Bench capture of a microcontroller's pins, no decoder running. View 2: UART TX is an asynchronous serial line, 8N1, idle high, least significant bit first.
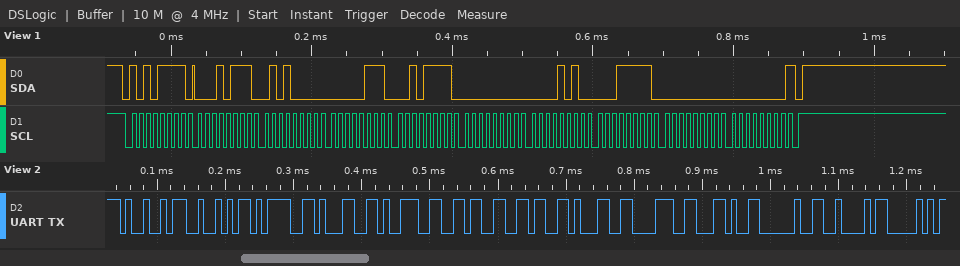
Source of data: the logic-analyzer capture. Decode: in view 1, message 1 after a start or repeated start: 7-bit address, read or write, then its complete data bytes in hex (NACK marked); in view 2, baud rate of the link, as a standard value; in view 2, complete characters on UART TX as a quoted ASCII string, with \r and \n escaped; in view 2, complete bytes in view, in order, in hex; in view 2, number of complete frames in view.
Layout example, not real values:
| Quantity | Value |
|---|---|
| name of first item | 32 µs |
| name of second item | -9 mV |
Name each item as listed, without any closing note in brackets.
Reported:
| Quantity | Value |
|---|---|
| in view 1, message 1 after a start or repeated start: 7-bit address, read or write, then its complete data bytes in hex | 0x57 read: 17 50 07 2F 00 0A 1F 00 00 NACK |
| in view 2, baud rate of the link, as a standard value | 115200 baud |
| in view 2, complete characters on UART TX as a quoted ASCII string, with \r and \n escaped | "IR=196618, BP" |
| in view 2, complete bytes in view, in order, in hex | 49 52 3D 31 39 36 36 31 38 2C 20 42 50 |
| in view 2, number of complete frames in view | 13 |
